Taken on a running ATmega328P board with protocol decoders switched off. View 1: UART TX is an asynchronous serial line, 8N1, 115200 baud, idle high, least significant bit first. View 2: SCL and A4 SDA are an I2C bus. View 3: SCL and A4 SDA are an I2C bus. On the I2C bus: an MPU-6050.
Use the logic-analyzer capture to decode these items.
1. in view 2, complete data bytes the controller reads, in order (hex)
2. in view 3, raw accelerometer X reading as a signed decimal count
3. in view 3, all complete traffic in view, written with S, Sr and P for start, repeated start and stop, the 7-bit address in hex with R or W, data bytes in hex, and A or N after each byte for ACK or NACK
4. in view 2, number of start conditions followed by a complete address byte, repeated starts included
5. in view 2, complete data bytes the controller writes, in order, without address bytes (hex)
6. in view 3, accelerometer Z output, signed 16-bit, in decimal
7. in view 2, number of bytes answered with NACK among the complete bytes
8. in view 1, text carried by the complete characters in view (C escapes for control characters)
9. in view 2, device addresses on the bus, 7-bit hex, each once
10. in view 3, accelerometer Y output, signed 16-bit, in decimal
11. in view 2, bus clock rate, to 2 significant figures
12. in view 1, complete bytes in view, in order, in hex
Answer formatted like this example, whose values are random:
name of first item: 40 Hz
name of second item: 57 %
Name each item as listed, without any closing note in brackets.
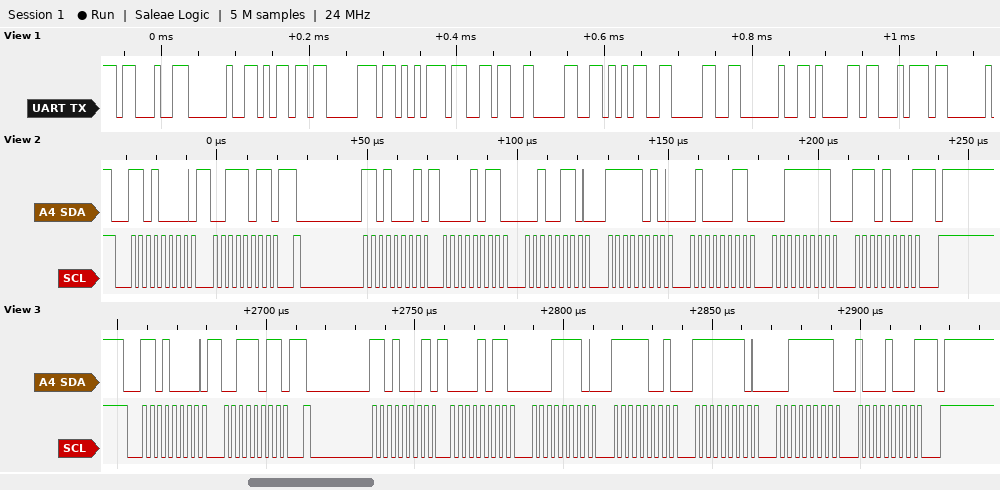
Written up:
in view 2, complete data bytes the controller reads, in order: 0B 26 FA 43 3F E8
in view 3, raw accelerometer X reading as a signed decimal count: 2846
in view 3, all complete traffic in view, written with S, Sr and P for start, repeated start and stop, the 7-bit address in hex with R or W, data bytes in hex, and A or N after each byte for ACK or NACK: S 68W A 3B A Sr 68R A 0B A 1E A F9 A FE A 3F A 88 N P
in view 2, number of start conditions followed by a complete address byte, repeated starts included: 2
in view 2, complete data bytes the controller writes, in order, without address bytes: 3B
in view 3, accelerometer Z output, signed 16-bit, in decimal: 16264
in view 2, number of bytes answered with NACK among the complete bytes: 1
in view 1, text carried by the complete characters in view: "# mpu6050 at"
in view 2, device addresses on the bus, 7-bit hex, each once: 0x68
in view 3, accelerometer Y output, signed 16-bit, in decimal: -1538
in view 2, bus clock rate, to 2 significant figures: 400 kHz
in view 1, complete bytes in view, in order, in hex: 23 20 6D 70 75 36 30 35 30 20 61 74
